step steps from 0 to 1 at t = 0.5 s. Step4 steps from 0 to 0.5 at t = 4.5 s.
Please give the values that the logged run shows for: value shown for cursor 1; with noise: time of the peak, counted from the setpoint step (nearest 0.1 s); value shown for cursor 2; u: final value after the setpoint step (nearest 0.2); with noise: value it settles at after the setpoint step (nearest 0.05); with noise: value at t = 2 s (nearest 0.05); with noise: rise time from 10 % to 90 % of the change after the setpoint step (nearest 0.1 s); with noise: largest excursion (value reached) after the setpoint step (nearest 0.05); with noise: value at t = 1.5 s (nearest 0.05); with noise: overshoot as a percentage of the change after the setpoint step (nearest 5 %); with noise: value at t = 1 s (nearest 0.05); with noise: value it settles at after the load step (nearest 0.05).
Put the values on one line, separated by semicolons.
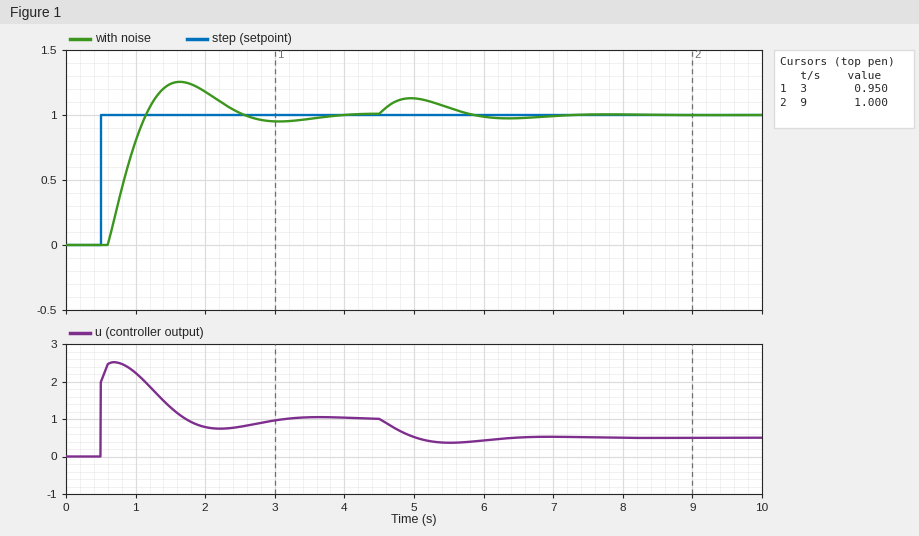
0.950; 1.1 s; 1.000; 1.0; 1.00; 1.20; 0.4 s; 1.25; 1.25; 25 %; 0.80; 1.00
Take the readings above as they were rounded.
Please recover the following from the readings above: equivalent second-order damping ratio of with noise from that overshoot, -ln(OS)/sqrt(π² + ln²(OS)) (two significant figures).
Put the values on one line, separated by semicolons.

0.40
